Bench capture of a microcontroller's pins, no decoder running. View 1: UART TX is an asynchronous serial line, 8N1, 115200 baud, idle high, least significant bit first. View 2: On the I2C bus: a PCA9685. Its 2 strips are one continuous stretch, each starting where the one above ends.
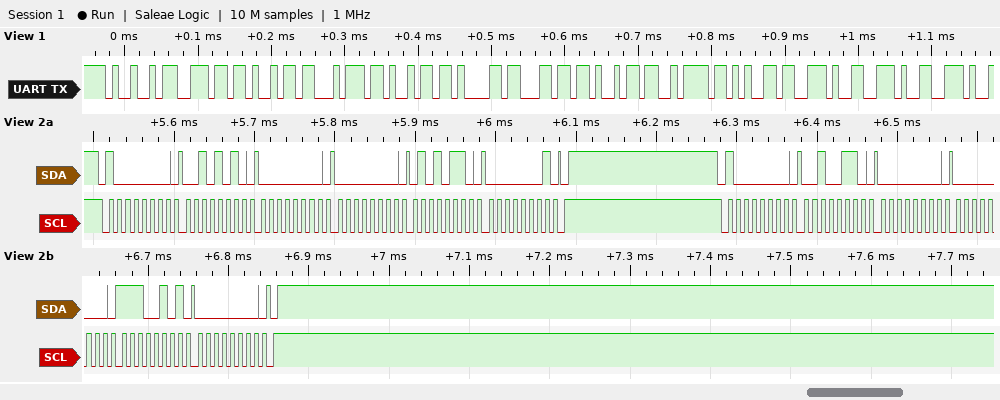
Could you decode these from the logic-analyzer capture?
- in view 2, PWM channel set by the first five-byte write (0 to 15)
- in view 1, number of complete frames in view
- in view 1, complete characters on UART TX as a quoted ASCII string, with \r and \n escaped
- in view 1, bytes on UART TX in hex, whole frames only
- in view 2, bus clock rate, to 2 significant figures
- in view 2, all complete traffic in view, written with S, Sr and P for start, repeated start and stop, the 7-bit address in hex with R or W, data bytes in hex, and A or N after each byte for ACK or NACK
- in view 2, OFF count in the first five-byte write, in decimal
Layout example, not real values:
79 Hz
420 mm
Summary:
9
13
"Initialize..."
49 6E 69 74 69 61 6C 69 7A 65 2E 2E 2E
100 kHz
S 40W A 2A A 00 A 00 A 56 A 01 A P S 40W A 26 A 00 A 00 A E5 A 00 A P
342
